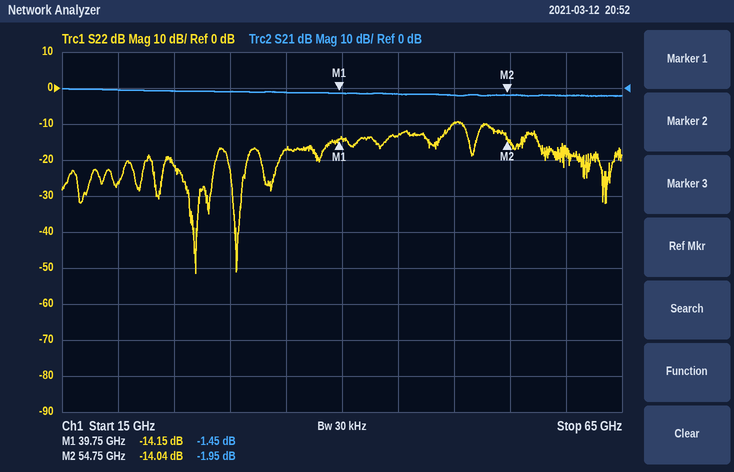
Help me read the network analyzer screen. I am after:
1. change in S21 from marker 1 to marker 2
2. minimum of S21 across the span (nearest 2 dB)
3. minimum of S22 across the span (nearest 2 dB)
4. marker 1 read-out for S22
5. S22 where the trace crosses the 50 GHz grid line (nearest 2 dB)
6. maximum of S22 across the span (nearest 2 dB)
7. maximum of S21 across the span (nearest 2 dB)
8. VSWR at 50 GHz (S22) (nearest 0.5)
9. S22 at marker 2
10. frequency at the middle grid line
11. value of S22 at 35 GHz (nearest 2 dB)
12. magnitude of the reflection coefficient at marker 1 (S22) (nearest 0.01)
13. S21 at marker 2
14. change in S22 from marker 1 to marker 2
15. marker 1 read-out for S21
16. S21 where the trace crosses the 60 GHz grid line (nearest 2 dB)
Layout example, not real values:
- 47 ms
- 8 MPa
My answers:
- -0.50 dB
- -2 dB
- -52 dB
- -14.15 dB
- -10 dB
- -10 dB
- 0 dB
- 2.0
- -14.04 dB
- 40 GHz
- -18 dB
- 0.20
- -1.95 dB
- 0.11 dB
- -1.45 dB
- -2 dB
